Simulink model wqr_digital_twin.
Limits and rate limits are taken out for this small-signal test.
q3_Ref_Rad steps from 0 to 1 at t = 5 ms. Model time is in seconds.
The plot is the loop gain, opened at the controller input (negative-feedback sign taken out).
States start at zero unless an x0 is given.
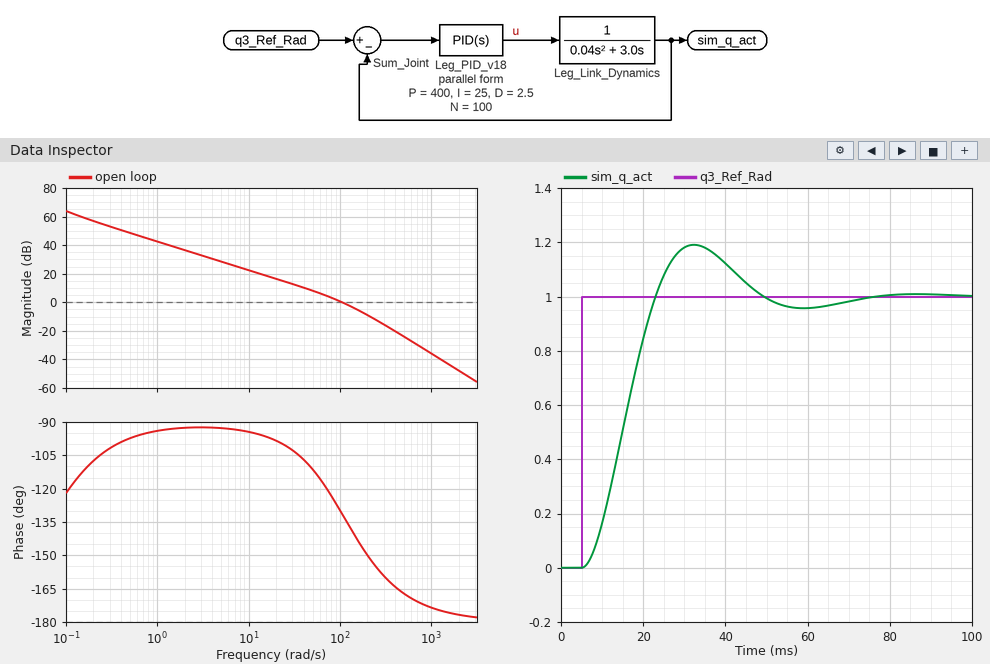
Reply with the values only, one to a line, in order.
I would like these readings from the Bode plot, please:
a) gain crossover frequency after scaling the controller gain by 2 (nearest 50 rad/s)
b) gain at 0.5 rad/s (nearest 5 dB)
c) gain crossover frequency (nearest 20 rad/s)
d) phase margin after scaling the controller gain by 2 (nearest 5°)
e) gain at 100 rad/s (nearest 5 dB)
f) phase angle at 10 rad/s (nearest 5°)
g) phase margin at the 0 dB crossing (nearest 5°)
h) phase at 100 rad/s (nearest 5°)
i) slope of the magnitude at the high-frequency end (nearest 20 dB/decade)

150 rad/s
50 dB
100 rad/s
35°
0 dB
-95°
50°
-130°
-40 dB/decade
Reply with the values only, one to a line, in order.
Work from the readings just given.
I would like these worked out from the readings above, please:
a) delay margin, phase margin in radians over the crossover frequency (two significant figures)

0.0087 s
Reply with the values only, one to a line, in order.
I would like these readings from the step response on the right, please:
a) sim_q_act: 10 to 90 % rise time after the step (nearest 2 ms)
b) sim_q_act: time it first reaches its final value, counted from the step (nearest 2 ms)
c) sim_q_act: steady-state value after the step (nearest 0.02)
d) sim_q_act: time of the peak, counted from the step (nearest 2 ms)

12 ms
18 ms
1.00
28 ms
